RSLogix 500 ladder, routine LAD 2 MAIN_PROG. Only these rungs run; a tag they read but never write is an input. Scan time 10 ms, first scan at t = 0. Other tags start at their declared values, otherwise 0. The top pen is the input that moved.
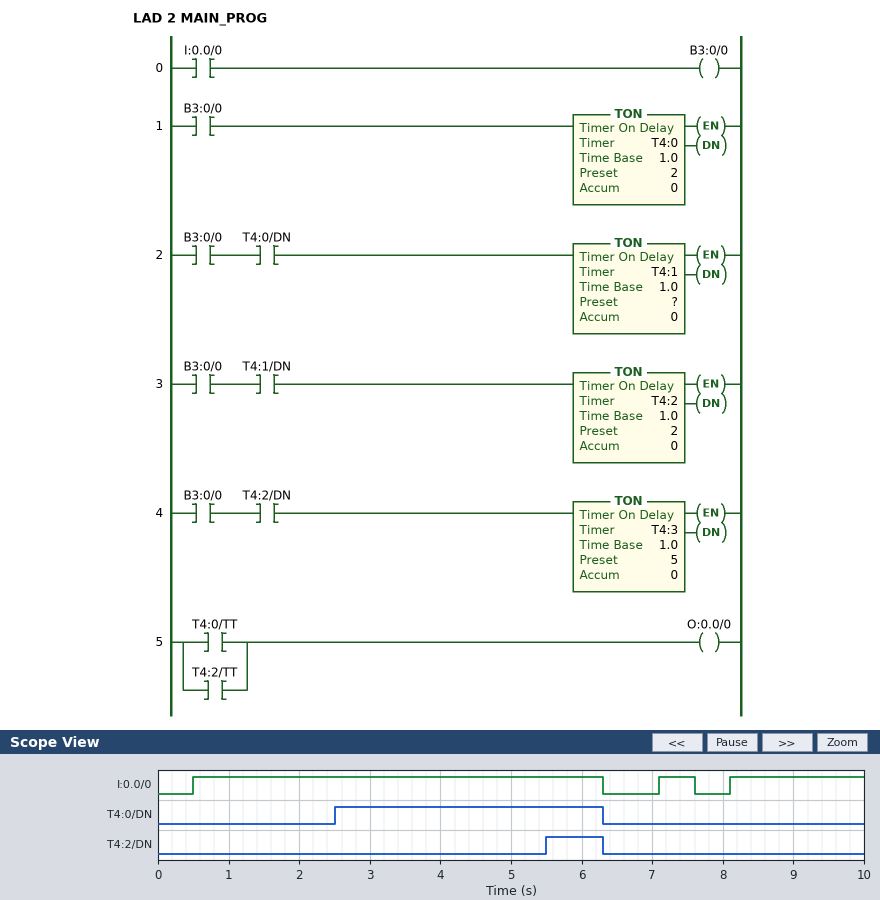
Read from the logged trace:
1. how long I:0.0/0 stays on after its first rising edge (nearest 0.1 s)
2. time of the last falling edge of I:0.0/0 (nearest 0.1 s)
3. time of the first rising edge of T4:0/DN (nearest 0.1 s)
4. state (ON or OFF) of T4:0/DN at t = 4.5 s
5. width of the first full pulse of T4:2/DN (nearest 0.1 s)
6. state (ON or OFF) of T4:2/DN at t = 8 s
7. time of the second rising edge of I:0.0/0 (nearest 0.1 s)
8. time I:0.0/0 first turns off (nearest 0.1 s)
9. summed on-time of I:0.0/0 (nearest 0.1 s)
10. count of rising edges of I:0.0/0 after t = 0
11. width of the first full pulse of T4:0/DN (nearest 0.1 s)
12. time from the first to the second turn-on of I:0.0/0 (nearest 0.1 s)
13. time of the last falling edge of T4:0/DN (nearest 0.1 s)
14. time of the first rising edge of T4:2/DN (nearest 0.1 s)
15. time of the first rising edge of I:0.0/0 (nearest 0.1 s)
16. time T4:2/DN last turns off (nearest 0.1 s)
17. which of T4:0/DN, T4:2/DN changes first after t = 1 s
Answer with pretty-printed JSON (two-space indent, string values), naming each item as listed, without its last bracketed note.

{
  "how long I:0.0/0 stays on after its first rising edge": "5.8 s",
  "time of the last falling edge of I:0.0/0": "7.6 s",
  "time of the first rising edge of T4:0/DN": "2.5 s",
  "state (ON or OFF) of T4:0/DN at t = 4.5 s": "ON",
  "width of the first full pulse of T4:2/DN": "0.8 s",
  "state (ON or OFF) of T4:2/DN at t = 8 s": "OFF",
  "time of the second rising edge of I:0.0/0": "7.1 s",
  "time I:0.0/0 first turns off": "6.3 s",
  "summed on-time of I:0.0/0": "8.2 s",
  "count of rising edges of I:0.0/0 after t = 0": "3",
  "width of the first full pulse of T4:0/DN": "3.8 s",
  "time from the first to the second turn-on of I:0.0/0": "6.6 s",
  "time of the last falling edge of T4:0/DN": "6.3 s",
  "time of the first rising edge of T4:2/DN": "5.5 s",
  "time of the first rising edge of I:0.0/0": "0.5 s",
  "time T4:2/DN last turns off": "6.3 s",
  "which of T4:0/DN, T4:2/DN changes first after t = 1 s": "T4:0/DN"
}
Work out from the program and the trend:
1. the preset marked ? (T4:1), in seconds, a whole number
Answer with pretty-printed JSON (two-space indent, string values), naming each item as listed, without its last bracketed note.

{
  "the preset marked ? (T4:1), in seconds, a whole number": "1 s"
}
